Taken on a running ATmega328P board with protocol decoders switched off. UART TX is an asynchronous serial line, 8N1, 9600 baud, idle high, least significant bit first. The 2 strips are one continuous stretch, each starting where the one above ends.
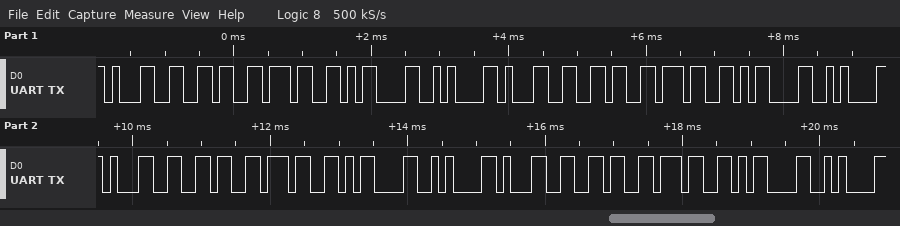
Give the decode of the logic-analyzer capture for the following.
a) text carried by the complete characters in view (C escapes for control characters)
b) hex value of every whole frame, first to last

"167\r\n167\r\n167\r\n167\r\n"
31 36 37 0D 0A 31 36 37 0D 0A 31 36 37 0D 0A 31 36 37 0D 0A
